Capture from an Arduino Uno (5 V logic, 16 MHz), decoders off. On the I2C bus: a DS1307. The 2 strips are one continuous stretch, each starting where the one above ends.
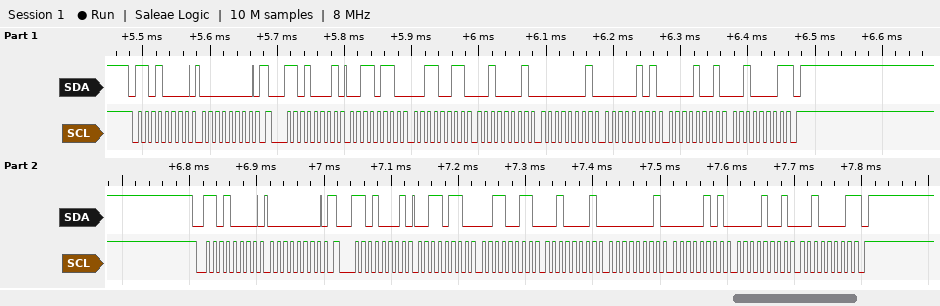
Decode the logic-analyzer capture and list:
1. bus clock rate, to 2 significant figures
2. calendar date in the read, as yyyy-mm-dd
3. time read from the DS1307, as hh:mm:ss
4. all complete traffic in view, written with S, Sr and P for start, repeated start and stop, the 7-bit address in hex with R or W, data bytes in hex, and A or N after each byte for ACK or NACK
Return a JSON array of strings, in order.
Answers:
["100 kHz", "2021-09-05", "21:33:36", "S 68W A 00 A Sr 68R A 36 A 33 A 21 A 01 A 05 A 09 A 21 N P S 68W A 00 A Sr 68R A 36 A 33 A 21 A 01 A 05 A 09 A 21 N P"]
